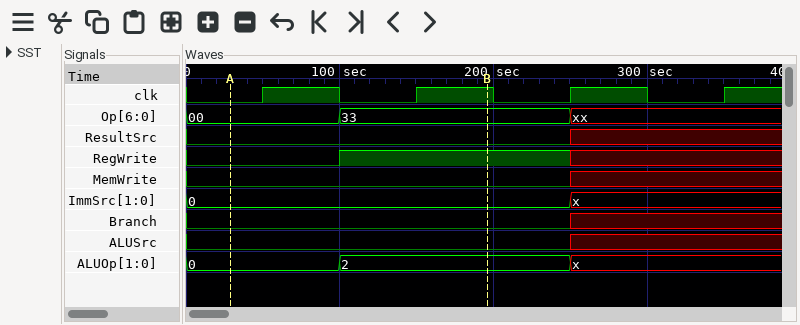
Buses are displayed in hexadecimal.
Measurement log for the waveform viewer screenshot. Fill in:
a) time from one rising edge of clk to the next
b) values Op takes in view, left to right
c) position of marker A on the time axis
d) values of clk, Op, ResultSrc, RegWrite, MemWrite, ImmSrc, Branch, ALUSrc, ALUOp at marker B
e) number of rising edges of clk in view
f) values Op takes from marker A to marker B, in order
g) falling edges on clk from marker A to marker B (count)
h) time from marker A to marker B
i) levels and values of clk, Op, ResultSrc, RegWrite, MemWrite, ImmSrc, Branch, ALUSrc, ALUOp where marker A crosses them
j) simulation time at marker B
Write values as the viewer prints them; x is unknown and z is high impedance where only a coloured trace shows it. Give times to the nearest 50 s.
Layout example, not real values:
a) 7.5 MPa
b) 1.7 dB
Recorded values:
a) 100 s
b) 00, 33, xx
c) 50 s
d) clk=1, Op=33, ResultSrc=0, RegWrite=1, MemWrite=0, ImmSrc=0, Branch=0, ALUSrc=0, ALUOp=2
e) 4
f) 00, 33
g) 1
h) 150 s
i) clk=0, Op=00, ResultSrc=0, RegWrite=0, MemWrite=0, ImmSrc=0, Branch=0, ALUSrc=0, ALUOp=0
j) 200 s
